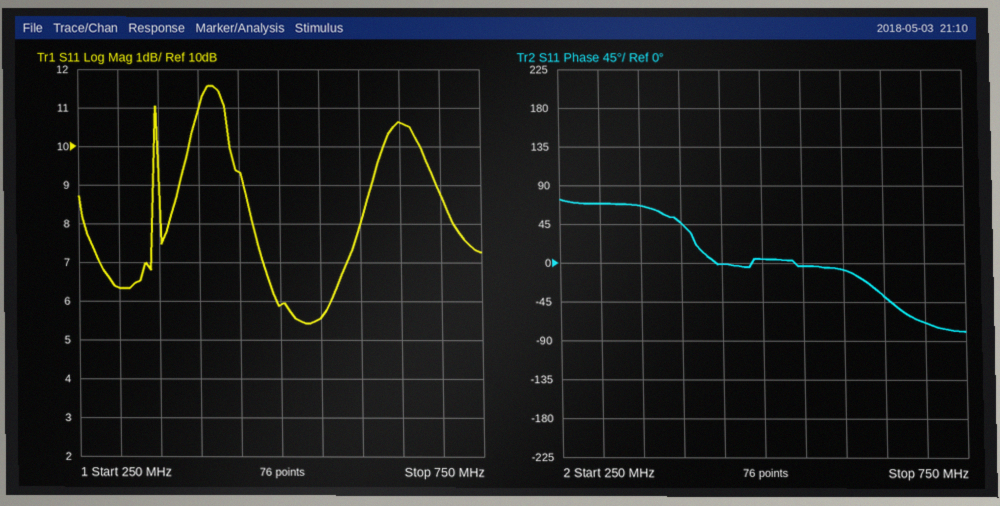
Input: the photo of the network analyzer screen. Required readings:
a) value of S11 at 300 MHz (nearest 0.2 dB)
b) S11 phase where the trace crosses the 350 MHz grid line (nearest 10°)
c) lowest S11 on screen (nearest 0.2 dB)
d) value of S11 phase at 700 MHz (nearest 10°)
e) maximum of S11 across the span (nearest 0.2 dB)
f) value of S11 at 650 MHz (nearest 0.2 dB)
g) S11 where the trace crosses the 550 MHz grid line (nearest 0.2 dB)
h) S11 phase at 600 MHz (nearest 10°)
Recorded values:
6.4 dB
70°
5.4 dB
-70°
11.6 dB
10.6 dB
5.6 dB
-10°
